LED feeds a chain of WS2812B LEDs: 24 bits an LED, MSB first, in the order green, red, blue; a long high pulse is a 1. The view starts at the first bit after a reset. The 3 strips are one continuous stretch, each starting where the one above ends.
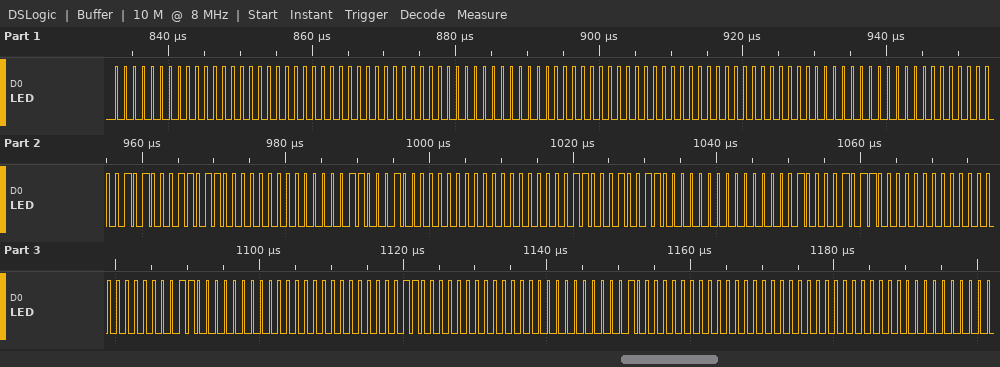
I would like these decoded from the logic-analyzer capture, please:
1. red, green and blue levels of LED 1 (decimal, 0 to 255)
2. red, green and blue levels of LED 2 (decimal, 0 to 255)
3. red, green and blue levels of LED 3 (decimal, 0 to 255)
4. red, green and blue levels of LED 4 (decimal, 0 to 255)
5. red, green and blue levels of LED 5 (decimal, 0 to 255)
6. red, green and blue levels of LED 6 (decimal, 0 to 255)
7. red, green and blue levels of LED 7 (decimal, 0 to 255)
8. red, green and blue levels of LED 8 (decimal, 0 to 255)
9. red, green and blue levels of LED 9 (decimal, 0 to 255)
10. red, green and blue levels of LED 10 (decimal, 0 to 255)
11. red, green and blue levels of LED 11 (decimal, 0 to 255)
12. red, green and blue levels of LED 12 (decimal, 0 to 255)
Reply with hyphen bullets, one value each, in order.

- 0, 0, 0
- 0, 0, 0
- 0, 0, 0
- 0, 0, 0
- 54, 10, 0
- 32, 6, 0
- 19, 3, 0
- 11, 1, 0
- 6, 0, 0
- 3, 0, 0
- 1, 0, 0
- 0, 0, 0
